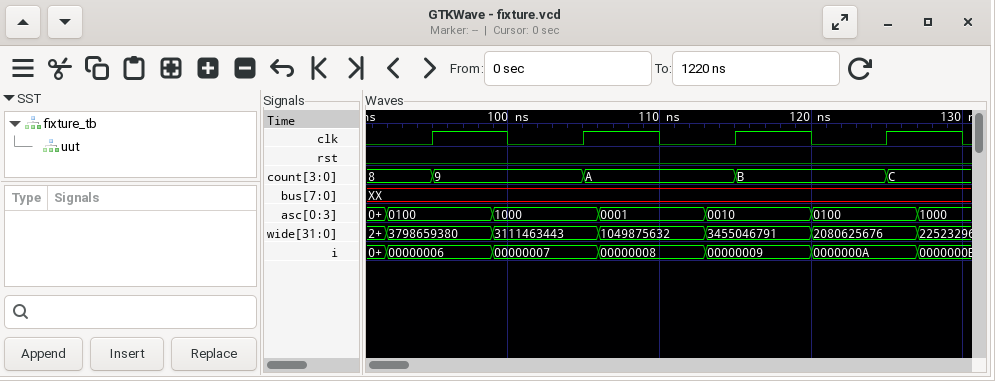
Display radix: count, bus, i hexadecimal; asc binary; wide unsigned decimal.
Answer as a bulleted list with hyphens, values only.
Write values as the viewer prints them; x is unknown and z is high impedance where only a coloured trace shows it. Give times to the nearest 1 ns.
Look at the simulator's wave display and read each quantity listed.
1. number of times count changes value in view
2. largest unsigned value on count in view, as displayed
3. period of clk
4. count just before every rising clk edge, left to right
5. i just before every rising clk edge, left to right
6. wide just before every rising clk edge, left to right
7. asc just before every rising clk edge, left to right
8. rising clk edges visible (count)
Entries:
- 4
- C
- 10 ns
- 8, 9, A, B
- 00000006, 00000007, 00000009, 0000000A
- 3798659380, 3111463443, 3455046791, 2080625676
- 0100, 1000, 0010, 0100
- 4
